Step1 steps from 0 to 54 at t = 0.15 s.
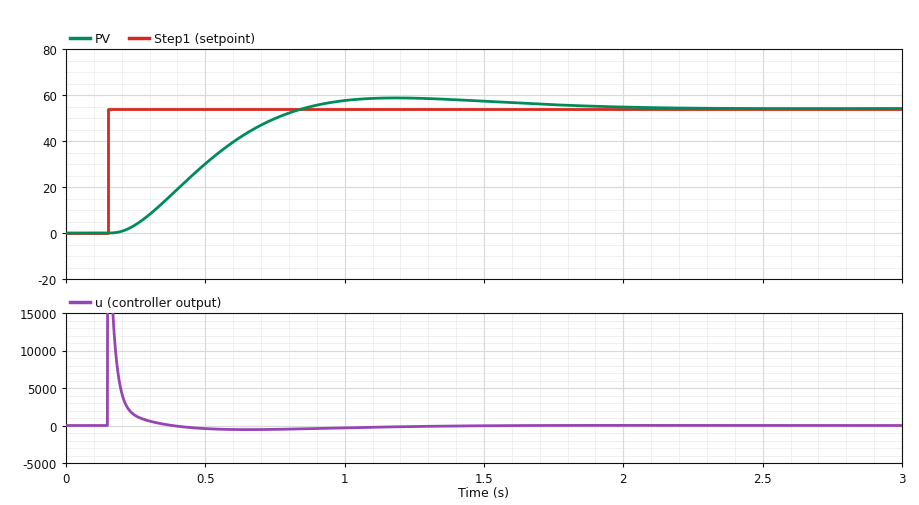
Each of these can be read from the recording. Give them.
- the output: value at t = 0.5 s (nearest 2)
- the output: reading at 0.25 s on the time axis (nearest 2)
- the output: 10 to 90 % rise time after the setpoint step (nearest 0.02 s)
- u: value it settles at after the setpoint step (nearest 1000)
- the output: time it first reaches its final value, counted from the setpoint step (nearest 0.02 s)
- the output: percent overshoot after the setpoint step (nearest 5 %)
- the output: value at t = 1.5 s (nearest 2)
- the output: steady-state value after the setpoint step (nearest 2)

30
4
0.46 s
0
0.70 s
10 %
58
54
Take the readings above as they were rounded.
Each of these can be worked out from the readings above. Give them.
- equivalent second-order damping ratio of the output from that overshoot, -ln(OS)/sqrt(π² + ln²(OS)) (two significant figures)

0.59
